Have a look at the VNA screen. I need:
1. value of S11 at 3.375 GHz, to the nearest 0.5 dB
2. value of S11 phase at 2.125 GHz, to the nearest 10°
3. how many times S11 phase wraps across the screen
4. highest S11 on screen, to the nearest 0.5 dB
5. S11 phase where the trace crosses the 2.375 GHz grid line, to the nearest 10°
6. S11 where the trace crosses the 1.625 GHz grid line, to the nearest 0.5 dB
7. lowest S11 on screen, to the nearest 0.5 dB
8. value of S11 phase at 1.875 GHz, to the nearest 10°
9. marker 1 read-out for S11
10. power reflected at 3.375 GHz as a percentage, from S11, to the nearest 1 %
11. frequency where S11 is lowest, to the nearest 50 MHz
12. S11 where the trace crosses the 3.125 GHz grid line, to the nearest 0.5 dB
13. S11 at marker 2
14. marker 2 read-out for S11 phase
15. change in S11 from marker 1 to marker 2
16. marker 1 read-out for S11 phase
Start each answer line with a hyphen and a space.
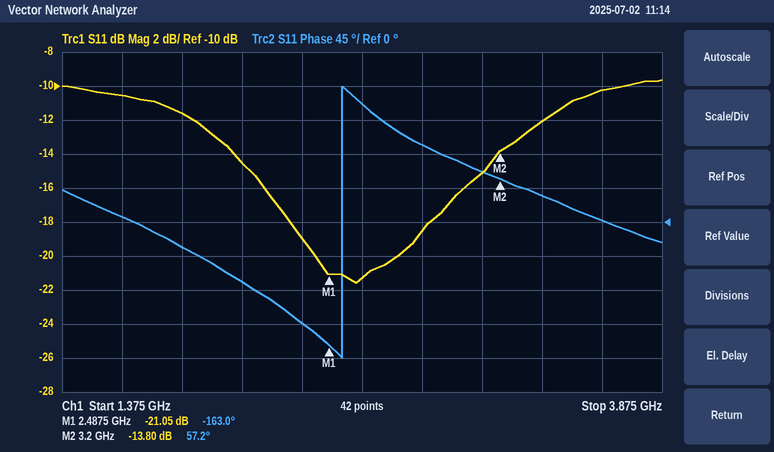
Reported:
- -12.0 dB
- -80°
- 1
- -9.5 dB
- -130°
- -10.5 dB
- -21.5 dB
- -30°
- -21.05 dB
- 6 %
- 2.60 GHz
- -15.0 dB
- -13.80 dB
- 57.2°
- 7.25 dB
- -163.0°
